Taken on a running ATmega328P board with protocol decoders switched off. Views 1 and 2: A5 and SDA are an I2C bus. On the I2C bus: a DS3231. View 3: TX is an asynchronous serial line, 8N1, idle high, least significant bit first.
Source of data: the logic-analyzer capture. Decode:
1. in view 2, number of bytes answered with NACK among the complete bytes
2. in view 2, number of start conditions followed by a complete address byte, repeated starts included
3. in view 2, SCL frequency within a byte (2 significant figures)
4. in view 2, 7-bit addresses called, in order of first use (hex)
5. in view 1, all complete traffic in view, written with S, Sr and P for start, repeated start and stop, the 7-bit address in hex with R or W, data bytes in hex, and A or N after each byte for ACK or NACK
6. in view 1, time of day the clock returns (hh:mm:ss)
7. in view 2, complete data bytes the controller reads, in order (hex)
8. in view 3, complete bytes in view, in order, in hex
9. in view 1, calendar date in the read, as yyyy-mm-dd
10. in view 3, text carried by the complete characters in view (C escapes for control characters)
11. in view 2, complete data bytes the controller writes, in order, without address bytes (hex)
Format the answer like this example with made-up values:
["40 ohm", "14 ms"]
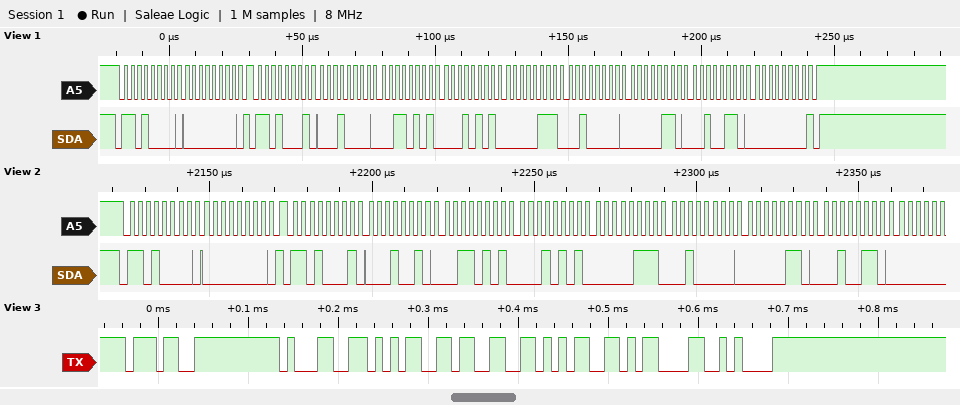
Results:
["0", "2", "400 kHz", "0x68", "S 68W A 00 A Sr 68R A 10 A 35 A 15 A 07 A 20 A 06 A 26 A 00 N P", "15:35:10", "12 35 15 07 20 06 26", "37 31 35 33 35 0D 0A", "2026-06-20", "\"71535\\r\\n\"", "00"]
